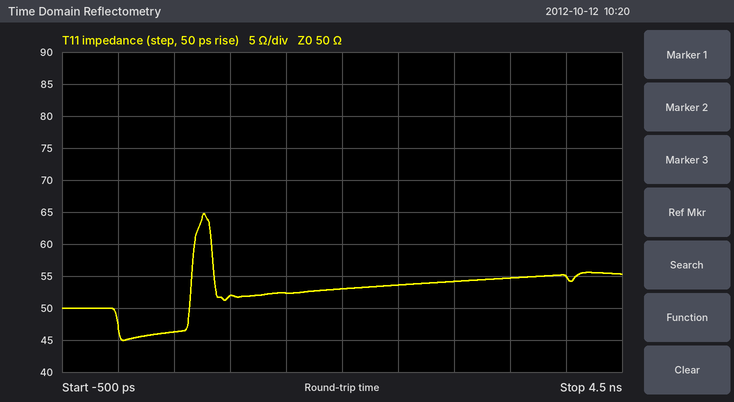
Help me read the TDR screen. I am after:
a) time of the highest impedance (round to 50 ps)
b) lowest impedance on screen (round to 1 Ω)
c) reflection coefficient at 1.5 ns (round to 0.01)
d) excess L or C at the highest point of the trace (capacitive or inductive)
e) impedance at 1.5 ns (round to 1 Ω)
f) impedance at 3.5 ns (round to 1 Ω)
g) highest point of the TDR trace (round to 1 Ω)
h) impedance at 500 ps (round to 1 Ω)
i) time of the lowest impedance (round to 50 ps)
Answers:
750 ps
45 Ω
+0.02
inductive
52 Ω
55 Ω
65 Ω
46 Ω
50 ps
